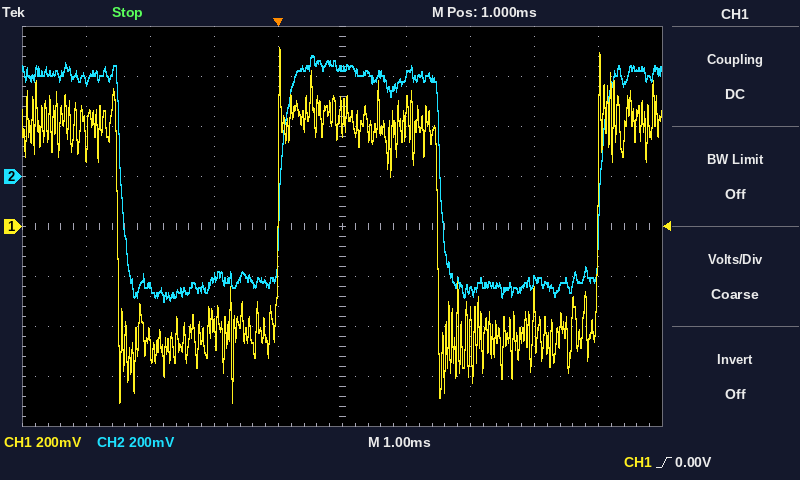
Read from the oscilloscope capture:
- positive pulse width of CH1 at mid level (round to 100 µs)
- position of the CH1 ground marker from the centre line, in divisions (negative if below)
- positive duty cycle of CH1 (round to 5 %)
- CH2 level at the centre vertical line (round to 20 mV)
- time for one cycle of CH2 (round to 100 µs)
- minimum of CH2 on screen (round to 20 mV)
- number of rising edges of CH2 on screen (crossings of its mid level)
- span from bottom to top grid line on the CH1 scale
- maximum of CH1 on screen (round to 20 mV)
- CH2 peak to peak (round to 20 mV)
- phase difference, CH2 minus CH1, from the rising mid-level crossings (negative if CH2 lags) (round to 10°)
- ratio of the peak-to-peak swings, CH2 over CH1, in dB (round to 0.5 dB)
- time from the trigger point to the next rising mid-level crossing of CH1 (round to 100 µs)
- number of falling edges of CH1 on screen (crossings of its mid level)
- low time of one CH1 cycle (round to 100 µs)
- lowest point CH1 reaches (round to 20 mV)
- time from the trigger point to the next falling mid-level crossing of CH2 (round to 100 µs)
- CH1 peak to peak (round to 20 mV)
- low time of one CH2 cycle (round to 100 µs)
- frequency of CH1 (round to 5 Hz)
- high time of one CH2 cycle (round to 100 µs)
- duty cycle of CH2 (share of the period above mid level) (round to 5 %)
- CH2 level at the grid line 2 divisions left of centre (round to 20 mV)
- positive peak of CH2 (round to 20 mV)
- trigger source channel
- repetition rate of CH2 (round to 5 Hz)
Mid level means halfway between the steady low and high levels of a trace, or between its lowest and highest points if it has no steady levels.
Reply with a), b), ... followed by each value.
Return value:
a) 2.5 ms
b) 0.0 div
c) 50 %
d) 440 mV
e) 5.0 ms
f) -500 mV
g) 2
h) 1.6 V
i) 720 mV
j) 980 mV
k) 0°
l) -3.0 dB
m) 5.0 ms
n) 2
o) 2.5 ms
p) -700 mV
q) 2.5 ms
r) 1.42 V
s) 2.5 ms
t) 200 Hz
u) 2.5 ms
v) 50 %
w) -400 mV
x) 480 mV
y) CH1
z) 200 Hz
